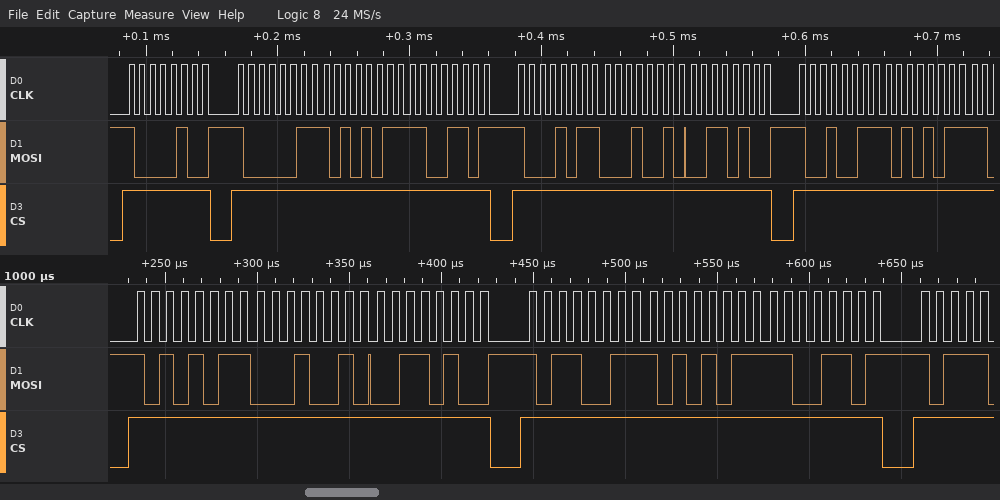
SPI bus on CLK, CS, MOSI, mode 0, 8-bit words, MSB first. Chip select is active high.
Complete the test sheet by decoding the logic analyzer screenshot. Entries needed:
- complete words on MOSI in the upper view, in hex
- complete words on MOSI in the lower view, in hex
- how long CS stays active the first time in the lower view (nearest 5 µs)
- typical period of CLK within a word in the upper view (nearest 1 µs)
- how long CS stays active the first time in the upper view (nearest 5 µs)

84, 83, AB, CD, 8B, 12, 34, 93, AB
AB, 12, 34, B3, AB, CD
195 µs
8 µs
65 µs
